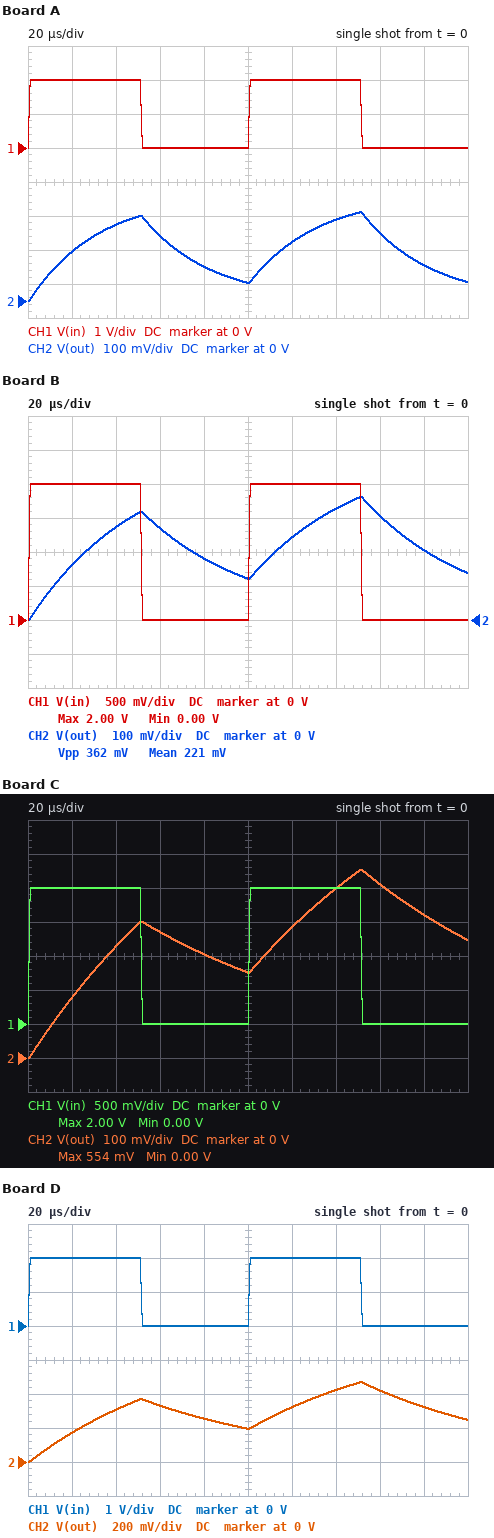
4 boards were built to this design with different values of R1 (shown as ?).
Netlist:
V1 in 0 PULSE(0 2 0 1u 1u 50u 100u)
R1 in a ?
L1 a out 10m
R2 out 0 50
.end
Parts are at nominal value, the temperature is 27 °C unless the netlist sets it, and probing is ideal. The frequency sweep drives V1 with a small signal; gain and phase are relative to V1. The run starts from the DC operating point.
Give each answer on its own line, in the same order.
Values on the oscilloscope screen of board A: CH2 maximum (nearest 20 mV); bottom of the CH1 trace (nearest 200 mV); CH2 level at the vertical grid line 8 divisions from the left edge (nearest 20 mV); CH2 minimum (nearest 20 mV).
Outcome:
260 mV
0 V
200 mV
0 V
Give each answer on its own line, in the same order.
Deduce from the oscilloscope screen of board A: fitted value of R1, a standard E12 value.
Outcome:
270 Ω
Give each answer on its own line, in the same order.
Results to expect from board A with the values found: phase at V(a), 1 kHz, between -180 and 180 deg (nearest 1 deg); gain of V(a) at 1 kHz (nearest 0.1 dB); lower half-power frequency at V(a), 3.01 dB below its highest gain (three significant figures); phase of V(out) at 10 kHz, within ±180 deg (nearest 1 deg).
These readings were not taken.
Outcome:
40 deg
-12.2 dB
4.97 kHz
-63 deg
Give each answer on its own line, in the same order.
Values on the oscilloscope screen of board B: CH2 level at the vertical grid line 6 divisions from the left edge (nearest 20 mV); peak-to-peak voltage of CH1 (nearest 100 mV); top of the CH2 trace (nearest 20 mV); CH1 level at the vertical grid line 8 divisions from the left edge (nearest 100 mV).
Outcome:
240 mV
2.0 V
360 mV
0 V
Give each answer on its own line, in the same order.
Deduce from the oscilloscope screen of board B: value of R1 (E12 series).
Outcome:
150 Ω
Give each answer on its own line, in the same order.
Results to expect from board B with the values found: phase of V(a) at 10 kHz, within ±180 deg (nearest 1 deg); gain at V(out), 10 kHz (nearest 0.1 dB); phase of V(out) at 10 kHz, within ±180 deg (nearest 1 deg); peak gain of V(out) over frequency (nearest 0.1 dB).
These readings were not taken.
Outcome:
13 deg
-22.4 dB
-72 deg
-12.0 dB
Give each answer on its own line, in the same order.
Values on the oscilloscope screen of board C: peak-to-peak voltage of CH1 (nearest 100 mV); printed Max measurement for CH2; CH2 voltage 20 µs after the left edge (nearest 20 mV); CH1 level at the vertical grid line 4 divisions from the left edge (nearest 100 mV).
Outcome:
2.0 V
554 mV
180 mV
0 V
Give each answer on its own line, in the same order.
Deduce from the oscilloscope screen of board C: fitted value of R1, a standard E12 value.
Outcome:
47 Ω
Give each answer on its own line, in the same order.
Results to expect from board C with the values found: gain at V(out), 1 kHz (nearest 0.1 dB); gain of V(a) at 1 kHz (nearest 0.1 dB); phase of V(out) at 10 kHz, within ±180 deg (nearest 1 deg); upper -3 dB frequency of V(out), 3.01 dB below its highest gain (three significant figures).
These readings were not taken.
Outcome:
-7.3 dB
-3.2 dB
-81 deg
1.54 kHz
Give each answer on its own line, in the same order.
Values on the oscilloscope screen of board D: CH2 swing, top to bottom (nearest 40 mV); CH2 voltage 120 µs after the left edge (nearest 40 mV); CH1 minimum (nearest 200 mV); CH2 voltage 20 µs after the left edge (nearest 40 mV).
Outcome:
480 mV
320 mV
0 V
160 mV
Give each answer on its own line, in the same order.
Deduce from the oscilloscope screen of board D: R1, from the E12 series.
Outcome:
82 Ω
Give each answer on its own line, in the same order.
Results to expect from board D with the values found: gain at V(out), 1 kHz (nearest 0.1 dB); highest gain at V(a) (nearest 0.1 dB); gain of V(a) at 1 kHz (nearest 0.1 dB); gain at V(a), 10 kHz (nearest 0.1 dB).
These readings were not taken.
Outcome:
-9.3 dB
0 dB
-5.2 dB
-0.2 dB
